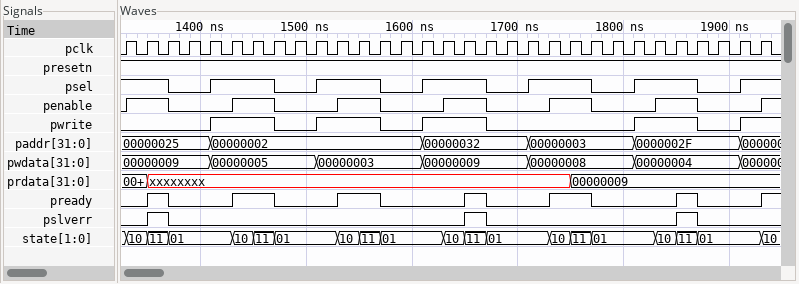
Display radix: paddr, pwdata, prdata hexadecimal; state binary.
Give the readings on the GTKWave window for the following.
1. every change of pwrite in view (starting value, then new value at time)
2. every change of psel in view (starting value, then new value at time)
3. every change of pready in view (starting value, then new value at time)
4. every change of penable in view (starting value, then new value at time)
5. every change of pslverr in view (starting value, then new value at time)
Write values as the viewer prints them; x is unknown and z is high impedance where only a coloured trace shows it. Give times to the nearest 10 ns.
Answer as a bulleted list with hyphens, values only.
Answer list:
- 0, 1 at 1410 ns, 0 at 1470 ns, 1 at 1510 ns, 0 at 1570 ns, 1 at 1610 ns, 0 at 1670 ns, 1 at 1810 ns, 0 at 1870 ns, 1 at 1910 ns
- 1, 0 at 1370 ns, 1 at 1410 ns, 0 at 1470 ns, 1 at 1510 ns, 0 at 1570 ns, 1 at 1610 ns, 0 at 1670 ns, 1 at 1710 ns, 0 at 1770 ns, 1 at 1810 ns, 0 at 1870 ns, 1 at 1910 ns
- 0, 1 at 1350 ns, 0 at 1370 ns, 1 at 1430 ns, 0 at 1470 ns, 1 at 1530 ns, 0 at 1570 ns, 1 at 1650 ns, 0 at 1670 ns, 1 at 1730 ns, 0 at 1770 ns, 1 at 1850 ns, 0 at 1870 ns, 1 at 1930 ns
- 0, 1 at 1330 ns, 0 at 1370 ns, 1 at 1430 ns, 0 at 1470 ns, 1 at 1530 ns, 0 at 1570 ns, 1 at 1630 ns, 0 at 1670 ns, 1 at 1730 ns, 0 at 1770 ns, 1 at 1830 ns, 0 at 1870 ns, 1 at 1930 ns
- 0, 1 at 1350 ns, 0 at 1370 ns, 1 at 1650 ns, 0 at 1670 ns, 1 at 1850 ns, 0 at 1870 ns
